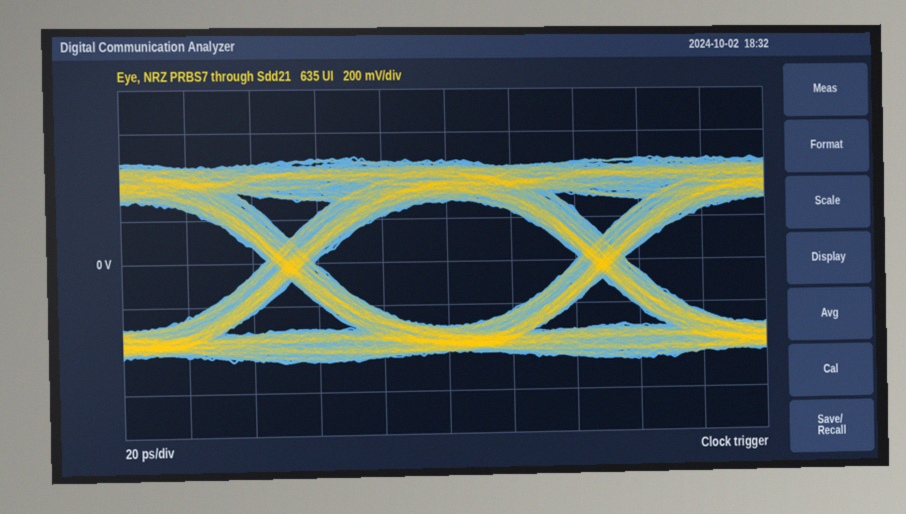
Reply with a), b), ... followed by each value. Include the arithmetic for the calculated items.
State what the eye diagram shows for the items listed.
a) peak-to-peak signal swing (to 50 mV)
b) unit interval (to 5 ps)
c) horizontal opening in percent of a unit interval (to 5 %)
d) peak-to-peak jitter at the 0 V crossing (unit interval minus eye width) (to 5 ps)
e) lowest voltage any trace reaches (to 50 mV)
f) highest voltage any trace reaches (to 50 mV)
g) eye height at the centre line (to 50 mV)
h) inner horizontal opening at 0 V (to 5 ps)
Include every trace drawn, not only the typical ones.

a) 950 mV
b) 95 ps
c) 80 ps / 95 ps ≈ 84.2 %, so 85 % to the nearest 5 %
d) 15 ps
e) -450 mV
f) 500 mV
g) 600 mV
h) 80 ps
